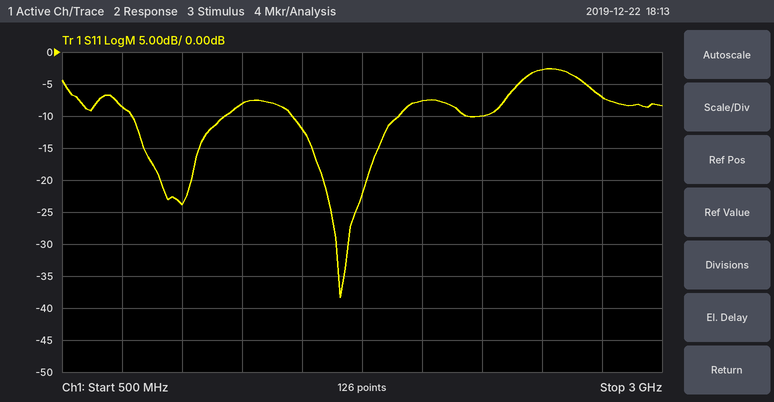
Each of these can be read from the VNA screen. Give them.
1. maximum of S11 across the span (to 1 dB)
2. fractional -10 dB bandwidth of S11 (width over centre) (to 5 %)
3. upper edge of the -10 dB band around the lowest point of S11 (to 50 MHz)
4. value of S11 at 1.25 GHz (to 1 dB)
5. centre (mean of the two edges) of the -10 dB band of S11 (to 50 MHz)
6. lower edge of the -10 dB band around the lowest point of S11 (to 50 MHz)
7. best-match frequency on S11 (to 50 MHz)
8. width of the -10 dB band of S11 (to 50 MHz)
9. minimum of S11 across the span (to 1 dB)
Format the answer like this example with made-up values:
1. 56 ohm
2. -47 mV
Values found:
1. -3 dB
2. 25 %
3. 1.90 GHz
4. -8 dB
5. 1.70 GHz
6. 1.45 GHz
7. 1.65 GHz
8. 450 MHz
9. -38 dB
